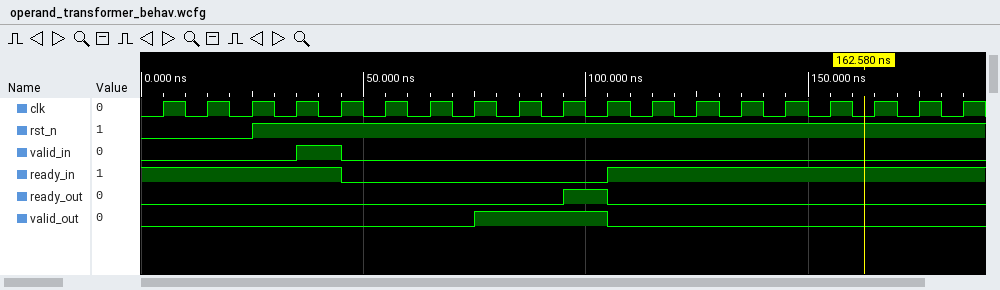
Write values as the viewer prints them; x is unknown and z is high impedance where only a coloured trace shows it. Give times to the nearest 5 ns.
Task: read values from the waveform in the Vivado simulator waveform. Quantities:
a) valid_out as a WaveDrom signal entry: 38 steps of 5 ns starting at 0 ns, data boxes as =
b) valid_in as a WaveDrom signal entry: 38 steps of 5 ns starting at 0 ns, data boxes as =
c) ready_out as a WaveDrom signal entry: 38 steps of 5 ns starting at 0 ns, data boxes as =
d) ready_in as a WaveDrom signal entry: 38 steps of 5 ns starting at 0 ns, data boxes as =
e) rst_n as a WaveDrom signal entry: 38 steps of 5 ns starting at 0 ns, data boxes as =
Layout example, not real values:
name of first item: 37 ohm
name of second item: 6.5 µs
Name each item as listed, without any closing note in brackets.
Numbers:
valid_out as a WaveDrom signal entry: 38 steps of 5 ns starting at 0 ns, data boxes as =: {name: 'valid_out', wave: '0..............1.....0................'}
valid_in as a WaveDrom signal entry: 38 steps of 5 ns starting at 0 ns, data boxes as =: {name: 'valid_in', wave: '0......1.0............................'}
ready_out as a WaveDrom signal entry: 38 steps of 5 ns starting at 0 ns, data boxes as =: {name: 'ready_out', wave: '0..................1.0................'}
ready_in as a WaveDrom signal entry: 38 steps of 5 ns starting at 0 ns, data boxes as =: {name: 'ready_in', wave: '1........0...........1................'}
rst_n as a WaveDrom signal entry: 38 steps of 5 ns starting at 0 ns, data boxes as =: {name: 'rst_n', wave: '0....1................................'}
